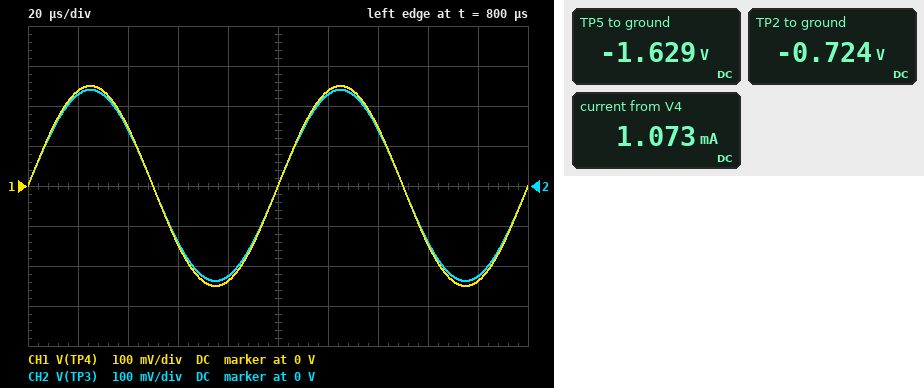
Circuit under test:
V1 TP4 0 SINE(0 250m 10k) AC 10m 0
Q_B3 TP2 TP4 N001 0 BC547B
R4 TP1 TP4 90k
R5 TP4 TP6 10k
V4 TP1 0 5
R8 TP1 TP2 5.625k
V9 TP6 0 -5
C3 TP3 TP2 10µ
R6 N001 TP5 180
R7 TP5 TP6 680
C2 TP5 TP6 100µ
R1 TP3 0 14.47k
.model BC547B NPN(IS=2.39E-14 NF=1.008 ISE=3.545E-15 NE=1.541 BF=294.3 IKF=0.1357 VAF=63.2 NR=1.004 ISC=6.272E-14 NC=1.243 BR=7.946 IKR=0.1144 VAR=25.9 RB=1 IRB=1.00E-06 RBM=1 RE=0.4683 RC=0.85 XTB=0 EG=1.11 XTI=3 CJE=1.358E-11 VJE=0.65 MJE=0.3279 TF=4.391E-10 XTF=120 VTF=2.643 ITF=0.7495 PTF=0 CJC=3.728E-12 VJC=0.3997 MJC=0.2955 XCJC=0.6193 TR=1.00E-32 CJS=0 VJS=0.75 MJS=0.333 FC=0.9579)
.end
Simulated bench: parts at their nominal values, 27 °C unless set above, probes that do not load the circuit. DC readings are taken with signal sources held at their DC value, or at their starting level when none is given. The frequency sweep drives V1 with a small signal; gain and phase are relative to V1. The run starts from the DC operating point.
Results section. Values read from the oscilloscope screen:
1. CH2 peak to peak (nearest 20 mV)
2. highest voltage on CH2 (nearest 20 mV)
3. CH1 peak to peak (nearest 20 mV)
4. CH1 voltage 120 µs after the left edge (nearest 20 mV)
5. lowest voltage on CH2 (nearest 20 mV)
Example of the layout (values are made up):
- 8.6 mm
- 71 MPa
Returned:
- 480 mV
- 240 mV
- 500 mV
- 240 mV
- -240 mV
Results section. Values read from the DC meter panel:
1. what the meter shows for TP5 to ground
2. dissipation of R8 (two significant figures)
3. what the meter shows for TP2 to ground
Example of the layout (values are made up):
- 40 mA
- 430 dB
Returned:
- -1.629 V
- 5.8 mW
- -0.724 V
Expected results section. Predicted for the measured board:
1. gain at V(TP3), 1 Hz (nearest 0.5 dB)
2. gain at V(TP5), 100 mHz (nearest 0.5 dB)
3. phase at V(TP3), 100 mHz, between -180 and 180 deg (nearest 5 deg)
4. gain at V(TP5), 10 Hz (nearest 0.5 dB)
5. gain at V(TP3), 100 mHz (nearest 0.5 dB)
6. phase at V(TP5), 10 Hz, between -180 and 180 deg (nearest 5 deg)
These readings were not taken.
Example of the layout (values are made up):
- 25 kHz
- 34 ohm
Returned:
- -3.5 dB
- -2.0 dB
- 85 deg
- -5.0 dB
- -21.0 dB
- -45 deg
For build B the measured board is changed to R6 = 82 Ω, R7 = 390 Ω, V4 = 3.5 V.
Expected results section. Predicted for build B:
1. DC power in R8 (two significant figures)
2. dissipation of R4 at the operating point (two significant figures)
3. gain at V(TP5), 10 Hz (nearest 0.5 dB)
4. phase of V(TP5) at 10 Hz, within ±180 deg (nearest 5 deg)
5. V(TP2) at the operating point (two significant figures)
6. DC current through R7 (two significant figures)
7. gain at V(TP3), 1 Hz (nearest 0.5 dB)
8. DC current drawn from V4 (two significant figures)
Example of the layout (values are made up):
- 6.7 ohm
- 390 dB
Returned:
- 3.2 mW
- 140 µW
- -2.5 dB
- -25 deg
- -750 mV
- 9.0 mA
- -3.5 dB
- 790 µA
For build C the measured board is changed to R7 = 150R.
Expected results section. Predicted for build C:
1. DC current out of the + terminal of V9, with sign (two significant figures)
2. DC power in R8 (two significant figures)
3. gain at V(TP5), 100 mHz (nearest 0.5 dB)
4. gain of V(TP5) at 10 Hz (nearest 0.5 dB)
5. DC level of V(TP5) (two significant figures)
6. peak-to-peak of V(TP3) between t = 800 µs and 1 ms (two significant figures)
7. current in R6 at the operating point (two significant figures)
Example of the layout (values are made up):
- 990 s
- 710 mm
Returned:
- -13 mA
- 5.9 mW
- -7.0 dB
- -8.0 dB
- -3.1 V
- 490 mV
- 13 mA
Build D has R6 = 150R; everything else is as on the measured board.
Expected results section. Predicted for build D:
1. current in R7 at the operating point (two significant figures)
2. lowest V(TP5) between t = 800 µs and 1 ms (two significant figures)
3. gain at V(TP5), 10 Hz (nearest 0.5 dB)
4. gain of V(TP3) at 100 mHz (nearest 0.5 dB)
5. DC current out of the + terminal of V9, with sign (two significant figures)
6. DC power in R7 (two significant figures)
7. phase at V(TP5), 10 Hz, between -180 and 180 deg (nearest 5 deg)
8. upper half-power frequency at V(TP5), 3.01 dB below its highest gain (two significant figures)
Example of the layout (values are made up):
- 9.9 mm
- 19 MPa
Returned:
- 5.1 mA
- -1.5 V
- -4.0 dB
- -21.0 dB
- -5.6 mA
- 18 mW
- -40 deg
- 12 Hz
